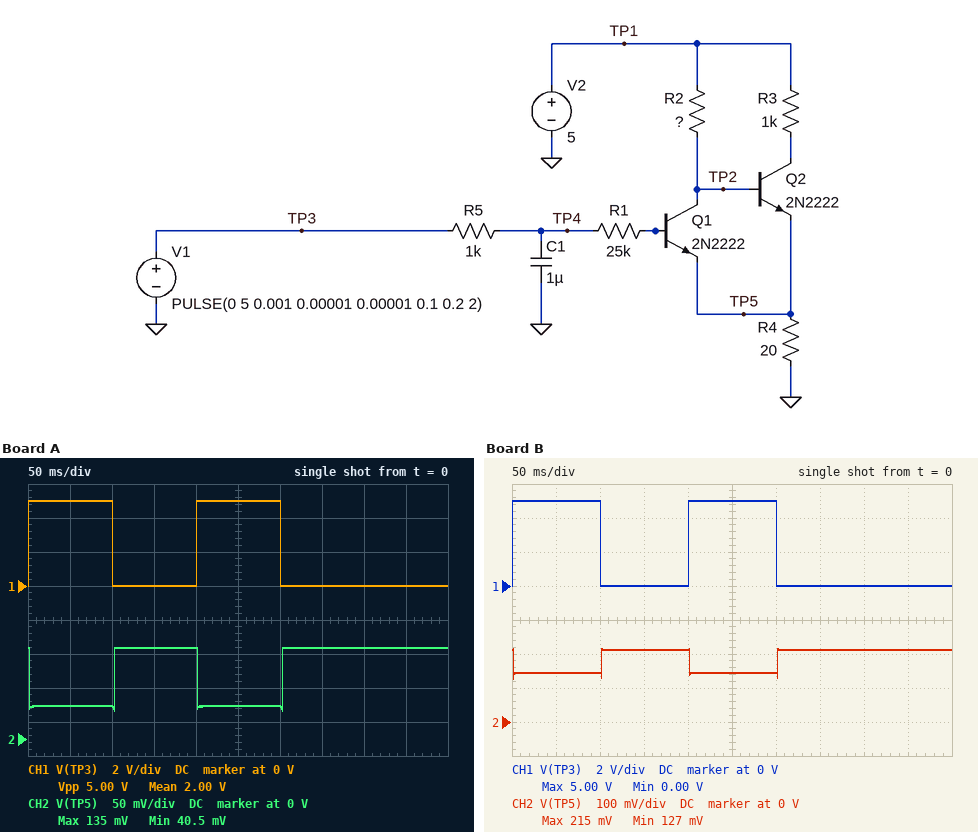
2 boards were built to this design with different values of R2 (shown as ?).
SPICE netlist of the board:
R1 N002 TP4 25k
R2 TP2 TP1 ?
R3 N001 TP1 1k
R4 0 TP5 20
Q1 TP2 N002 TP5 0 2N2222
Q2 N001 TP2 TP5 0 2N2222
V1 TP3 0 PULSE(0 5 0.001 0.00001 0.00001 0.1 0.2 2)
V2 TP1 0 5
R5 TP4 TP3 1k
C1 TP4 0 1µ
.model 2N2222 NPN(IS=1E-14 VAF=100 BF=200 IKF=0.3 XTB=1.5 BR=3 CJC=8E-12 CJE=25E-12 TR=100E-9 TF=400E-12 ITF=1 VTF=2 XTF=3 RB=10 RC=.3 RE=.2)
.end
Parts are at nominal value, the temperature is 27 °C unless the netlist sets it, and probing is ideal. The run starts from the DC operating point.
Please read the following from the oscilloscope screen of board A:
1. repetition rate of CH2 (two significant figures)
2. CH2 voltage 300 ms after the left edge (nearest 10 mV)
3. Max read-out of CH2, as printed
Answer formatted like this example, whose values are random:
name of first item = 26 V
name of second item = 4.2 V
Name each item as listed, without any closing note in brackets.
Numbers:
repetition rate of CH2 = 5.0 Hz
CH2 voltage 300 ms after the left edge = 50 mV
Max read-out of CH2, as printed = 135 mV
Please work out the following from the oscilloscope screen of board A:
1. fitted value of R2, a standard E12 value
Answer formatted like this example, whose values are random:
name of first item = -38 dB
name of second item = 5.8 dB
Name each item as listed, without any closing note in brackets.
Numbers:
fitted value of R2, a standard E12 value = 2.2 kΩ
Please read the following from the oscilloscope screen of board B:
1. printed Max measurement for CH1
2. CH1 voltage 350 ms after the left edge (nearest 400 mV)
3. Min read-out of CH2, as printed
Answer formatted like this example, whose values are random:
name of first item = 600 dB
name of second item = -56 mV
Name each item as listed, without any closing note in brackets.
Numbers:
printed Max measurement for CH1 = 5.00 V
CH1 voltage 350 ms after the left edge = 0 V
Min read-out of CH2, as printed = 127 mV
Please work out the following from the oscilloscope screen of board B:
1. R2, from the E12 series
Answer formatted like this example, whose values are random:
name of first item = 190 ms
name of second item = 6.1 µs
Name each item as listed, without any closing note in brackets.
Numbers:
R2, from the E12 series = 680 Ω
